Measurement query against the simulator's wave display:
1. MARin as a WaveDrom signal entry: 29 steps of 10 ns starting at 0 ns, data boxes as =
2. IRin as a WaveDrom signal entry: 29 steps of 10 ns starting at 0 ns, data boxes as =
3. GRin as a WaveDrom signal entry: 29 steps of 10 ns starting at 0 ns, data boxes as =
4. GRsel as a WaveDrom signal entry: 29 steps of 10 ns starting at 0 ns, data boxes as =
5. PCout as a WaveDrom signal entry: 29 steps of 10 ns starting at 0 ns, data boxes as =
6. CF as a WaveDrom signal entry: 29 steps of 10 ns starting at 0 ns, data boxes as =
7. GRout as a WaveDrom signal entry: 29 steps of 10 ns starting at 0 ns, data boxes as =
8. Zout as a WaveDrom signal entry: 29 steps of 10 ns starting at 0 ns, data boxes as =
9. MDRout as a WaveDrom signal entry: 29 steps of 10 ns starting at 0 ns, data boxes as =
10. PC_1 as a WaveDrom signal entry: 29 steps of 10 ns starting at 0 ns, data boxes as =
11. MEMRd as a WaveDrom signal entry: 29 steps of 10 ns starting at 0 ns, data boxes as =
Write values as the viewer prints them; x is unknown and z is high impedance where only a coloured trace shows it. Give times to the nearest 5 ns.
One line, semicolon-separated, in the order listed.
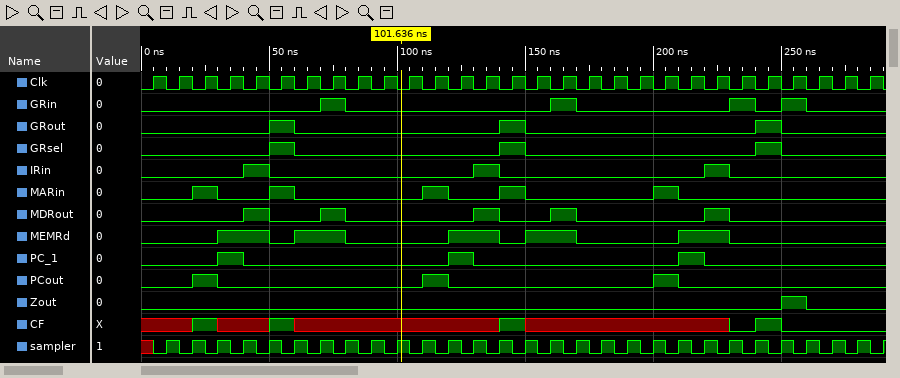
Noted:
{name: 'MARin', wave: '0.10.10....10.10....10.......'}; {name: 'IRin', wave: '0...10.......10.......10.....'}; {name: 'GRin', wave: '0......10.......10.....1010..'}; {name: 'GRsel', wave: '0....10.......10........10...'}; {name: 'PCout', wave: '0.10.......10.......10.......'}; {name: 'CF', wave: 'x.1x.1x.......1x.......010...'}; {name: 'GRout', wave: '0....10.......10........10...'}; {name: 'Zout', wave: '0........................10..'}; {name: 'MDRout', wave: '0...10.10....10.10....10.....'}; {name: 'PC_1', wave: '0..10.......10.......10......'}; {name: 'MEMRd', wave: '0..1.01.0...1.01.0...1.0.....'}
